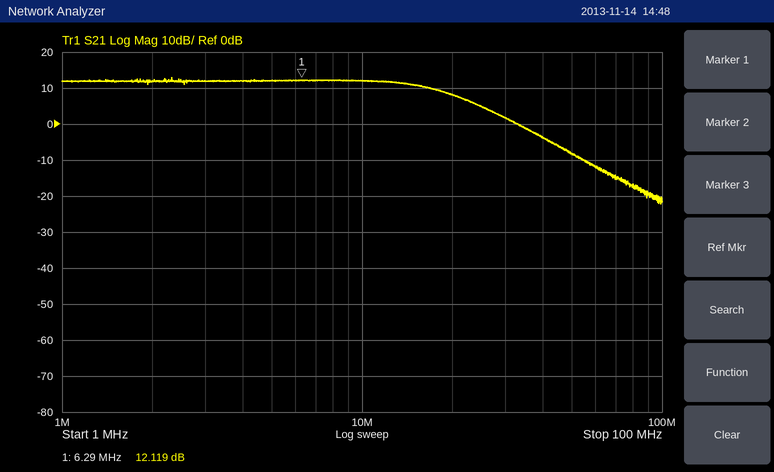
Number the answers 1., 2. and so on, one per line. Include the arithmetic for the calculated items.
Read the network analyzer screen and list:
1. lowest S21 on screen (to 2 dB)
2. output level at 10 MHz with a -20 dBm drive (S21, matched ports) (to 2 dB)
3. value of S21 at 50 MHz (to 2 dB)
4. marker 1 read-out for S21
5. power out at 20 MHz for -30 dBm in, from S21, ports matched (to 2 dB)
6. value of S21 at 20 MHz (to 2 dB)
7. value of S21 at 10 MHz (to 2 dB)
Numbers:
1. -22 dB
2. -20 dBm + (12 dB) = -8 dBm
3. -8 dB
4. 12.119 dB
5. -30 dBm + (8 dB) = -22 dBm
6. 8 dB
7. 12 dB
